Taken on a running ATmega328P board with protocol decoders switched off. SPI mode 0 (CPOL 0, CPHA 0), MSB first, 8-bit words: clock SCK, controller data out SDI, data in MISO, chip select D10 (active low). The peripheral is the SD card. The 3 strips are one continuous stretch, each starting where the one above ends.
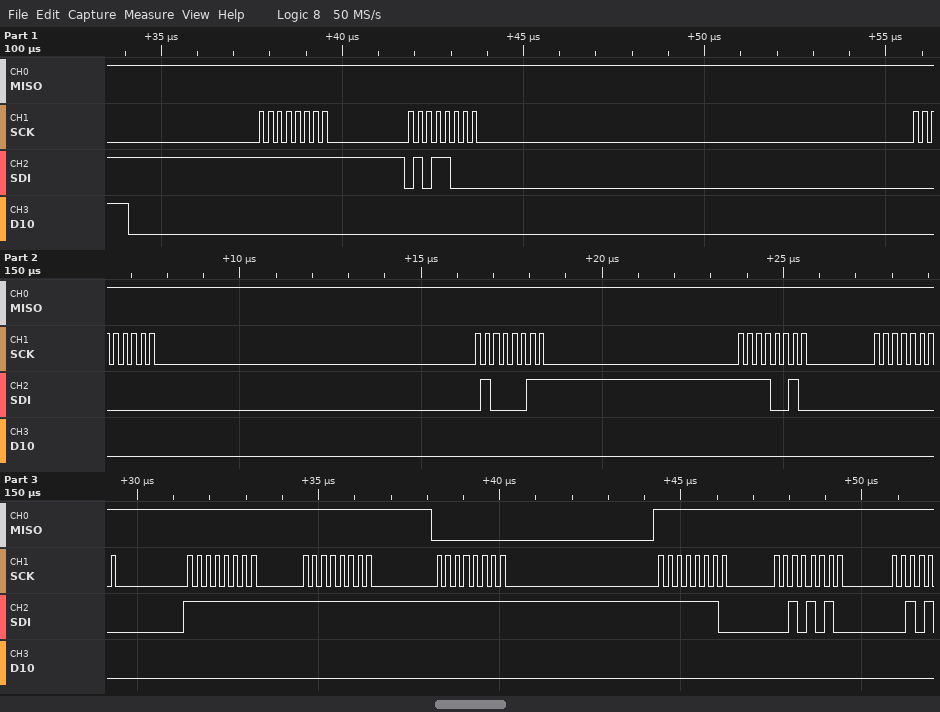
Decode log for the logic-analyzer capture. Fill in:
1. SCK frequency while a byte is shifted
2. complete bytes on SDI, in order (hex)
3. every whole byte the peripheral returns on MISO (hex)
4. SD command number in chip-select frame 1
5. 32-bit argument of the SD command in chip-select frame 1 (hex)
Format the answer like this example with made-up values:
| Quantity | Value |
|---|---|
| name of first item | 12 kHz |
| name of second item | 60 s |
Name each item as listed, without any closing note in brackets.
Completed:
| Quantity | Value |
|---|---|
| SCK frequency while a byte is shifted | 4 MHz |
| complete bytes on SDI, in order | FF 58 00 43 F2 00 FF FF FF FE 2A |
| every whole byte the peripheral returns on MISO | FF FF FF FF FF FF FF FF 00 FF FF |
| SD command number in chip-select frame 1 | CMD24 |
| 32-bit argument of the SD command in chip-select frame 1 | 0x0043F200 |
